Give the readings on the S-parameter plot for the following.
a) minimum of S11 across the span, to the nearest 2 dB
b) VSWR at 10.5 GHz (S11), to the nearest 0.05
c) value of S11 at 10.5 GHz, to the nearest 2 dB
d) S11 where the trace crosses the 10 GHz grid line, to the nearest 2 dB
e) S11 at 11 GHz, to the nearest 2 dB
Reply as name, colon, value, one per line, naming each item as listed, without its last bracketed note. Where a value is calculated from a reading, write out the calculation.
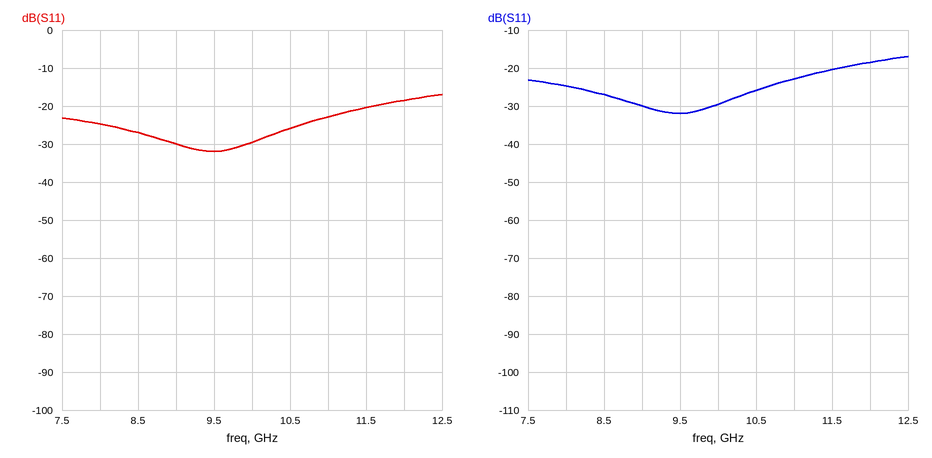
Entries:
minimum of S11 across the span, to the nearest 2 dB: -32 dB
VSWR at 10.5 GHz (S11), to the nearest 0.05: |Γ| = 10^(-26/20) = 0.0501; VSWR = (1 + 0.0501)/(1 − 0.0501) ≈ 1.11, so 1.10 to the nearest 0.05
value of S11 at 10.5 GHz, to the nearest 2 dB: -26 dB
S11 where the trace crosses the 10 GHz grid line, to the nearest 2 dB: -30 dB
S11 at 11 GHz, to the nearest 2 dB: -22 dB
